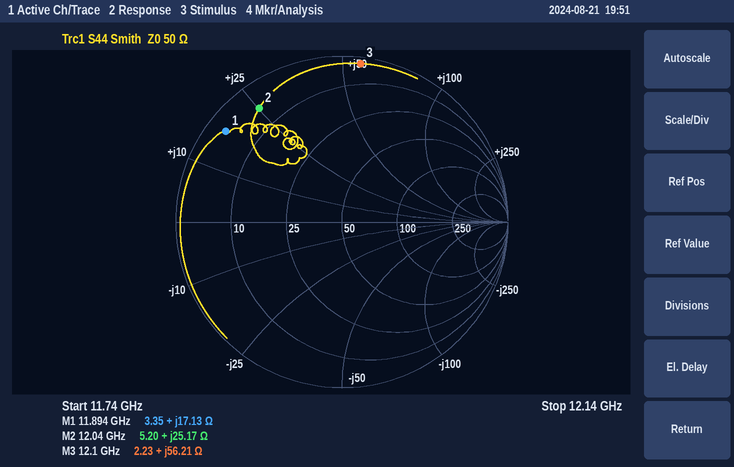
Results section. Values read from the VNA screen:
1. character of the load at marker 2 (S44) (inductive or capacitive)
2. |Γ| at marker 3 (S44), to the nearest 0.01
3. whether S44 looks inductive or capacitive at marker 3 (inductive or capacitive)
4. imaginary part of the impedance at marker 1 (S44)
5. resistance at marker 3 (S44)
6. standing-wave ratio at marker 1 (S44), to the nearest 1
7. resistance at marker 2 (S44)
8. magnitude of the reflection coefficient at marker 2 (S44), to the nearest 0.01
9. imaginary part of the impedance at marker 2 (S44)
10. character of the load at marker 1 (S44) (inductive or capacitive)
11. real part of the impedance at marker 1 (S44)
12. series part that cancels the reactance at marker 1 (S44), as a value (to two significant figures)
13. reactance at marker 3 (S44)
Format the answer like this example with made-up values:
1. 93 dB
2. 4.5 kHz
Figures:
1. inductive
2. 0.96
3. inductive
4. +17.13 Ω
5. 2.23 Ω
6. 17
7. 5.20 Ω
8. 0.85
9. +25.17 Ω
10. inductive
11. 3.35 Ω
12. 780 fF
13. +56.21 Ω
